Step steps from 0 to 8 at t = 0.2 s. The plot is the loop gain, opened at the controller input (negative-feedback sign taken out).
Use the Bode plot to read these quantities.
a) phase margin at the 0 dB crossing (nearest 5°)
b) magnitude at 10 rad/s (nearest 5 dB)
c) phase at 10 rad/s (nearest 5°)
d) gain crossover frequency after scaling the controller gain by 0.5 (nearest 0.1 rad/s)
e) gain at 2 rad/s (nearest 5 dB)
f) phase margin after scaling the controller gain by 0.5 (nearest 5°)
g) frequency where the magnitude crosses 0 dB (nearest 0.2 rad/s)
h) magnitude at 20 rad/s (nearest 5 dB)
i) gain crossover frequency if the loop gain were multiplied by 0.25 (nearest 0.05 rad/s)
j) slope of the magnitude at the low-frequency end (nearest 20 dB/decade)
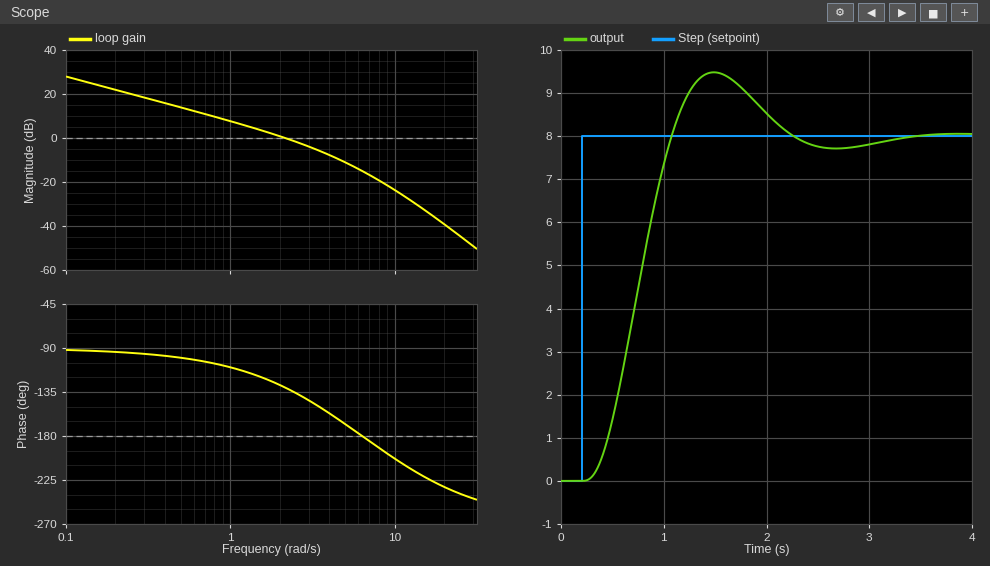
50°
-25 dB
-205°
1.2 rad/s
0 dB
65°
2.2 rad/s
-40 dB
0.60 rad/s
-20 dB/decade
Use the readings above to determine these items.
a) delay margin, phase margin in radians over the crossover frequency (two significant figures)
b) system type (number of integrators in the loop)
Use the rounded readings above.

0.40 s
1
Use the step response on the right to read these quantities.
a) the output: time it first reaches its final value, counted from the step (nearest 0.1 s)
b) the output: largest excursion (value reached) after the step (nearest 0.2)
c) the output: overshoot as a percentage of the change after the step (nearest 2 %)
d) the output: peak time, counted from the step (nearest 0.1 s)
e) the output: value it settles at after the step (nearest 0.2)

0.9 s
9.4
18 %
1.3 s
8.0
